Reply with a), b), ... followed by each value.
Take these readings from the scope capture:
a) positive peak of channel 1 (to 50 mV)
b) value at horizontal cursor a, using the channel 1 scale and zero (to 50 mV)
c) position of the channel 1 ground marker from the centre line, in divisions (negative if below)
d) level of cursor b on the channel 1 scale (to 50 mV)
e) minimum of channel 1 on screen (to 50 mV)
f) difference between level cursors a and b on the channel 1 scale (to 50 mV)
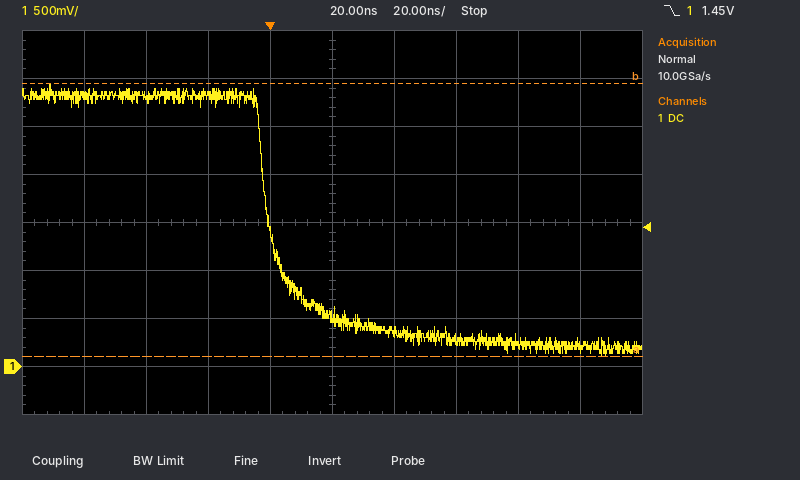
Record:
a) 2.95 V
b) 100 mV
c) -3.0 div
d) 2.95 V
e) 100 mV
f) 2.85 V
